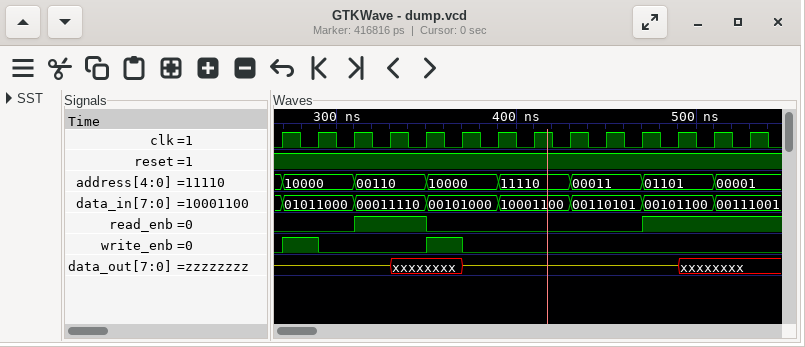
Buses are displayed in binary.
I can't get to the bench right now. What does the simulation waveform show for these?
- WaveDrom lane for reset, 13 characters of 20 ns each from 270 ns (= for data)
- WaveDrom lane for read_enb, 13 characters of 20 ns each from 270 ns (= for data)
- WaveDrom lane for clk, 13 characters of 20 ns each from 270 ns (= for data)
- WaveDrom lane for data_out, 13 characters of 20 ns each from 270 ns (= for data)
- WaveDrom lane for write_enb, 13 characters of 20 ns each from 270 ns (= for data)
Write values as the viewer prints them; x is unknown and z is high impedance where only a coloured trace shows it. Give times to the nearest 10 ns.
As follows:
{name: 'reset', wave: '1............'}
{name: 'read_enb', wave: '0.1.0.....1..'}
{name: 'clk', wave: 'p............'}
{name: 'data_out', wave: 'z..x.z.....x.'}
{name: 'write_enb', wave: '10..10.......'}
